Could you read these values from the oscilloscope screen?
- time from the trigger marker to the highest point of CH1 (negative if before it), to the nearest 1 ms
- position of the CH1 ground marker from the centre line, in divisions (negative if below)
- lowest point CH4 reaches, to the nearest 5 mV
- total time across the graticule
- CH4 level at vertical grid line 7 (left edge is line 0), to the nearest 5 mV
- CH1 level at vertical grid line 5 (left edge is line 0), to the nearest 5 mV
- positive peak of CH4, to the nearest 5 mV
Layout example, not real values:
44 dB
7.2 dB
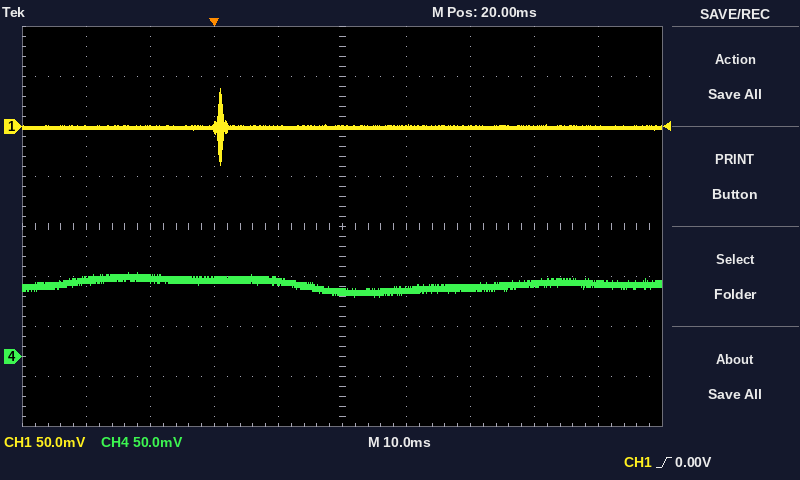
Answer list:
+1 ms
+2.0 div
60 mV
100 ms
70 mV
0 mV
85 mV
